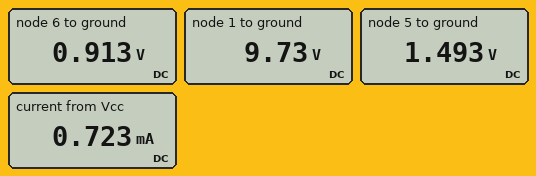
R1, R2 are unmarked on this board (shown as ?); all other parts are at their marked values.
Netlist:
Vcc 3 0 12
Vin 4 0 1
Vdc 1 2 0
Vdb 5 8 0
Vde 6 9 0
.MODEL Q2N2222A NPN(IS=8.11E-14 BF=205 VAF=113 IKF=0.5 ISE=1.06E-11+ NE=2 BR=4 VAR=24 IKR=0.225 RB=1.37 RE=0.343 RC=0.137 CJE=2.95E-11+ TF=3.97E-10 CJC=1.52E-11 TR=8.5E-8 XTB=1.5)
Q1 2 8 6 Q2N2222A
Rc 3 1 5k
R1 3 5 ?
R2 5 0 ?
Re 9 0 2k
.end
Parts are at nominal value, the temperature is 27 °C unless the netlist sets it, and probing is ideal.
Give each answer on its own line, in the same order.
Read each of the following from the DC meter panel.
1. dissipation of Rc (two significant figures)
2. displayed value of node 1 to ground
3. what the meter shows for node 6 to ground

1.0 mW
9.73 V
0.913 V
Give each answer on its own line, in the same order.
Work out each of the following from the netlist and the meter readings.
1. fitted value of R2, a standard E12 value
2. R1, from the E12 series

5.6 kΩ
39 kΩ
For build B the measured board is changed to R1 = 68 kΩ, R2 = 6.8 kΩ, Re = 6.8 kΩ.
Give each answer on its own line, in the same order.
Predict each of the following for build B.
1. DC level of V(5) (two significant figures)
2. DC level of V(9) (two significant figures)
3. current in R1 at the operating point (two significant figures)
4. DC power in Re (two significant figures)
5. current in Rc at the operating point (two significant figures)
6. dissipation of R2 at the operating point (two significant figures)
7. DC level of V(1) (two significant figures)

1.1 V
550 mV
160 µA
45 µW
81 µA
170 µW
12 V
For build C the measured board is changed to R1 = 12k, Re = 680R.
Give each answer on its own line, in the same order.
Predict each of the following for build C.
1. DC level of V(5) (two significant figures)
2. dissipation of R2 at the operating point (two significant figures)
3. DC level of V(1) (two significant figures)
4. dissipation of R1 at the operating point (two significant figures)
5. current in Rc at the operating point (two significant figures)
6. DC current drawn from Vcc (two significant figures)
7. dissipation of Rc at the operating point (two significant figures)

2.3 V
950 µW
1.7 V
7.8 mW
2.1 mA
2.9 mA
21 mW
